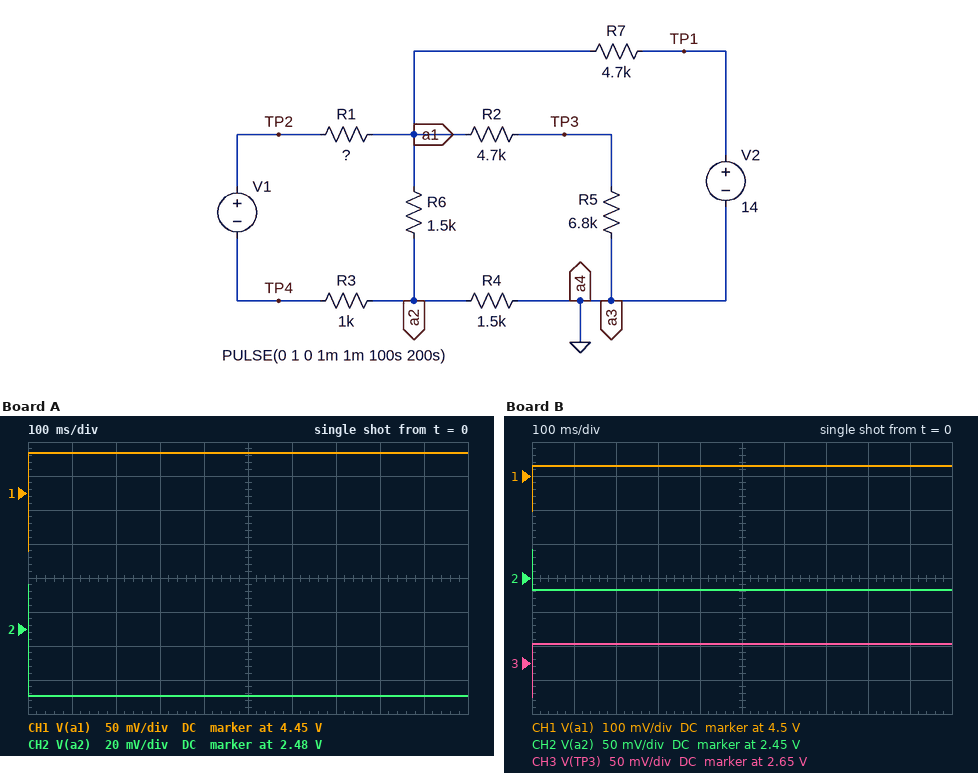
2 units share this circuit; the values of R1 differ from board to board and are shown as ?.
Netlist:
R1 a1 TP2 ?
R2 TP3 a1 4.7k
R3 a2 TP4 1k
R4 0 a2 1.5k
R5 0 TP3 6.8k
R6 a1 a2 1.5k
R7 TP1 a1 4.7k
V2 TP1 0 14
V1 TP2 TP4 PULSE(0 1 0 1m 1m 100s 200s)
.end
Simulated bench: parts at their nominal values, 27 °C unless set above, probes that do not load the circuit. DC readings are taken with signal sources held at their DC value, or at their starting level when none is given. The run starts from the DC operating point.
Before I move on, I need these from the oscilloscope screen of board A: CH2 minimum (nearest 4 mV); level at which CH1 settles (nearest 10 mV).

2.440 V
4.51 V
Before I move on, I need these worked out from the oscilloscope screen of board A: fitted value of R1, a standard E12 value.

3.3 kΩ
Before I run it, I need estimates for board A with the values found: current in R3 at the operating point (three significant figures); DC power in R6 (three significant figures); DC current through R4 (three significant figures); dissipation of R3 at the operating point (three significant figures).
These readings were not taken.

432 µA
2.30 mW
1.67 mA
187 µW
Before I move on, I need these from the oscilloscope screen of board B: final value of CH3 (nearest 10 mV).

2.68 V
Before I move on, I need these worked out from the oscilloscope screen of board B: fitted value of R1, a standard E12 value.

3.9 kΩ
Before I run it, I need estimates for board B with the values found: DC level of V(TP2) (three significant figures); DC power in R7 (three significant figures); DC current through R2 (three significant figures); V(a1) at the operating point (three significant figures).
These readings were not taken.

2.88 V
19.6 mW
382 µA
4.40 V
